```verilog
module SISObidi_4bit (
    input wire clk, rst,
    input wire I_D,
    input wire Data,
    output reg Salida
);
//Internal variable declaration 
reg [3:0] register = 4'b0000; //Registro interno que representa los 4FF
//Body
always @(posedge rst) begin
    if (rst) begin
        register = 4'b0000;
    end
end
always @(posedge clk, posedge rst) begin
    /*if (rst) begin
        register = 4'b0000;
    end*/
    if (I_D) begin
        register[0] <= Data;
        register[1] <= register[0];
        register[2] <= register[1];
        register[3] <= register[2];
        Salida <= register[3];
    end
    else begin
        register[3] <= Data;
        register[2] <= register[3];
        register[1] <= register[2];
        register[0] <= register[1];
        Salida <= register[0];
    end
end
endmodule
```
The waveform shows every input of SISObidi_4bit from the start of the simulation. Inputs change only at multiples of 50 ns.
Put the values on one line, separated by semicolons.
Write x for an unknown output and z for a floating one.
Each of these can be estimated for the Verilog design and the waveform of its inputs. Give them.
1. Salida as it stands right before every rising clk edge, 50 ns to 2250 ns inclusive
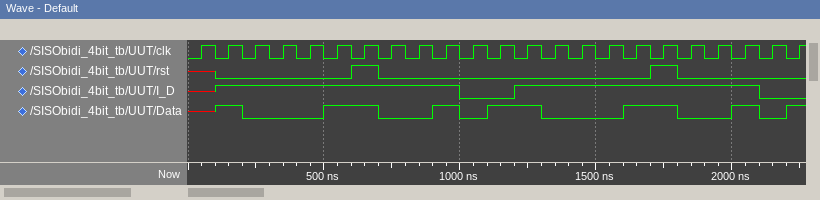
x 0 x 0 0 0 0 0 0 0 1 1 0 1 0 1 0 0 0 0 0 1 1
